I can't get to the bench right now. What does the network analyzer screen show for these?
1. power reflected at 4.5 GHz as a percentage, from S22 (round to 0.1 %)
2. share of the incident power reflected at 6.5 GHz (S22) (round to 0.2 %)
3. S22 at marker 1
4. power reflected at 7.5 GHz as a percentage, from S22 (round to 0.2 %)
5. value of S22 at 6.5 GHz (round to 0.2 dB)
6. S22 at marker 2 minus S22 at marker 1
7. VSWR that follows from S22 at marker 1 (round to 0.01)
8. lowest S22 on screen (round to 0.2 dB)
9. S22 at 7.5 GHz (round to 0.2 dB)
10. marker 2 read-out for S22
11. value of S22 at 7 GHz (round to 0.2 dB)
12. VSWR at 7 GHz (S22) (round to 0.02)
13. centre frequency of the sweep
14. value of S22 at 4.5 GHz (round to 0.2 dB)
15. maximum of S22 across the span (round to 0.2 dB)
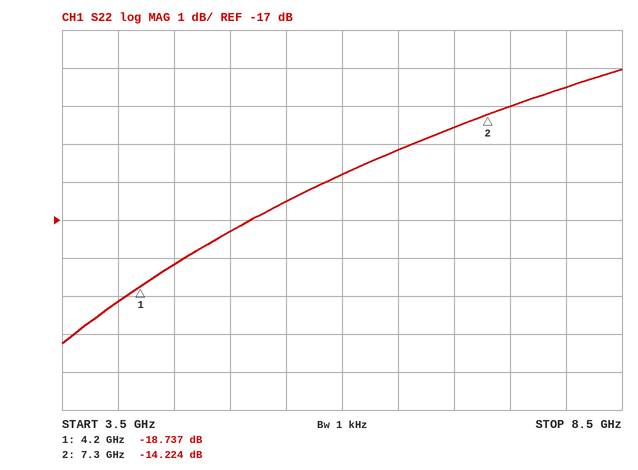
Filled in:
1.5 %
3.0 %
-18.737 dB
4.0 %
-15.2 dB
4.513 dB
1.26
-20.2 dB
-14.0 dB
-14.224 dB
-14.6 dB
1.46
6 GHz
-18.2 dB
-13.0 dB
